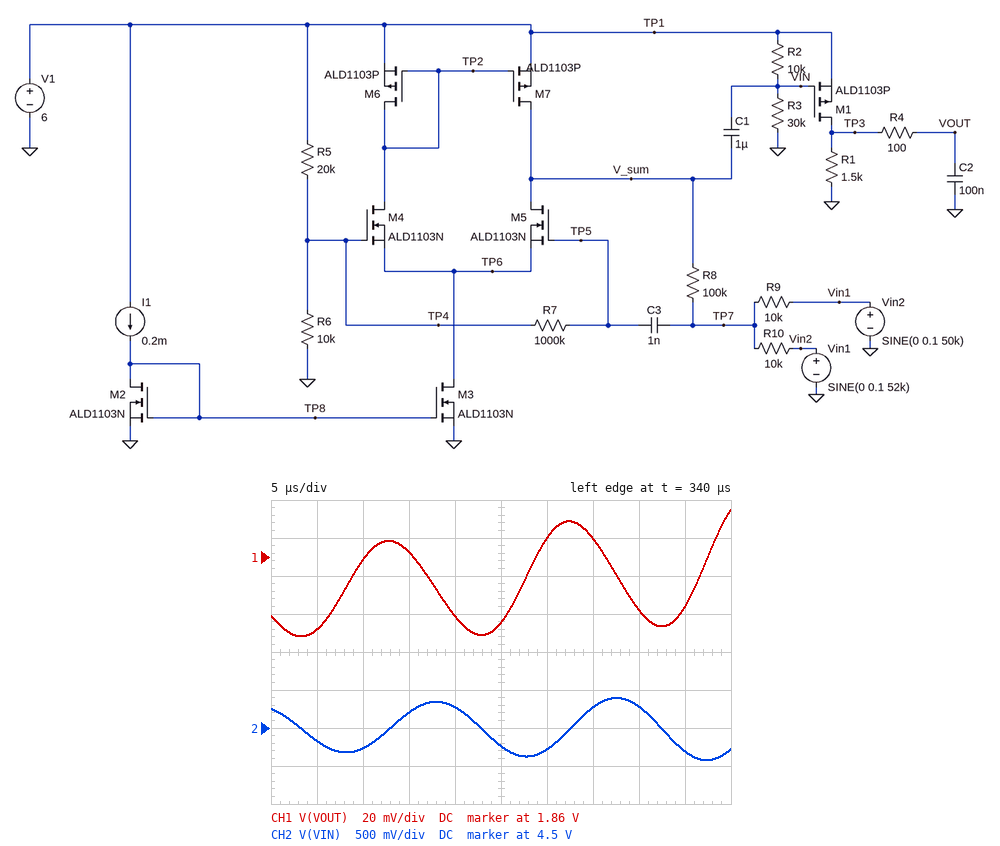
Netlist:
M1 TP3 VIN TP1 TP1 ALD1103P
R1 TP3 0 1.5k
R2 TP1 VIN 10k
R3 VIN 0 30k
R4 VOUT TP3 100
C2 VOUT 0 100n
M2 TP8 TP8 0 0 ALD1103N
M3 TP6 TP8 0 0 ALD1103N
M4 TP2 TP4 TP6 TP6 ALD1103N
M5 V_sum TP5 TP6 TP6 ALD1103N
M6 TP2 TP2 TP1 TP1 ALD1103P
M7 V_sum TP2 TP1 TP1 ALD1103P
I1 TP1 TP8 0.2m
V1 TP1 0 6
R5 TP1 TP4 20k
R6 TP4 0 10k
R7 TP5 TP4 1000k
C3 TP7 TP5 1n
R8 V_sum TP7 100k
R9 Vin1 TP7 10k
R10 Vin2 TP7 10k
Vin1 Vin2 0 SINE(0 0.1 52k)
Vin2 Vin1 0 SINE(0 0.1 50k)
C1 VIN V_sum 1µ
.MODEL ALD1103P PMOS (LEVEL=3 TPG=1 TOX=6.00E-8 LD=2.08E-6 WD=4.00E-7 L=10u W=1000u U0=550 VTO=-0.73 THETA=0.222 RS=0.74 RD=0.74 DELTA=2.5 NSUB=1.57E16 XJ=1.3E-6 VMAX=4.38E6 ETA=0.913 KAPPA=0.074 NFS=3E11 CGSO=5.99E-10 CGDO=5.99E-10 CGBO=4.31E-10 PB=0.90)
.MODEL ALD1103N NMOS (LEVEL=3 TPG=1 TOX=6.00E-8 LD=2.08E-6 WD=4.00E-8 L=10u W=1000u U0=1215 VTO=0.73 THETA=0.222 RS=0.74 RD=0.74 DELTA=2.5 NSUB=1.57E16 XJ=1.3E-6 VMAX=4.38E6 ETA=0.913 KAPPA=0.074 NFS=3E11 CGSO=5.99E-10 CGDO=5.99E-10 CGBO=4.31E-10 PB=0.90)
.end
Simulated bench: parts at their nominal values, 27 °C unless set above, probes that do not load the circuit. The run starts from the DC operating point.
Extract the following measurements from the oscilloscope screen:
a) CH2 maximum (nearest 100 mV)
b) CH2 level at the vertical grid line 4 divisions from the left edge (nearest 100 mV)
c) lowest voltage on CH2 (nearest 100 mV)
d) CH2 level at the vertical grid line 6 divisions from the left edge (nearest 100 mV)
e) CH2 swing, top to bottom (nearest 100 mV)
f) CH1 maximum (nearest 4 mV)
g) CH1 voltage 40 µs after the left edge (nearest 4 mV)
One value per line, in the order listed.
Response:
4.9 V
4.8 V
4.1 V
4.2 V
800 mV
1.884 V
1.832 V
